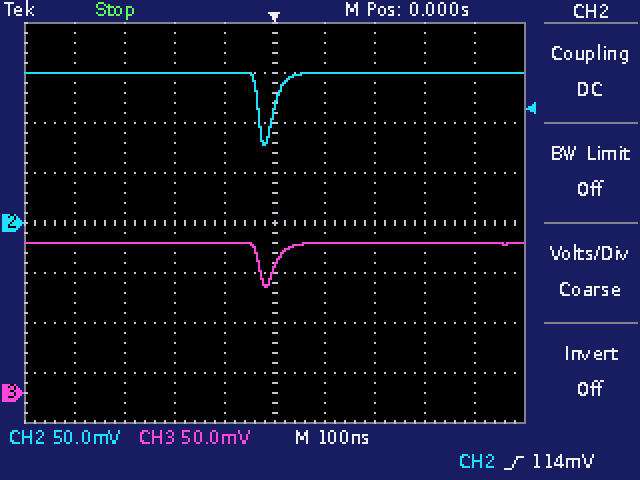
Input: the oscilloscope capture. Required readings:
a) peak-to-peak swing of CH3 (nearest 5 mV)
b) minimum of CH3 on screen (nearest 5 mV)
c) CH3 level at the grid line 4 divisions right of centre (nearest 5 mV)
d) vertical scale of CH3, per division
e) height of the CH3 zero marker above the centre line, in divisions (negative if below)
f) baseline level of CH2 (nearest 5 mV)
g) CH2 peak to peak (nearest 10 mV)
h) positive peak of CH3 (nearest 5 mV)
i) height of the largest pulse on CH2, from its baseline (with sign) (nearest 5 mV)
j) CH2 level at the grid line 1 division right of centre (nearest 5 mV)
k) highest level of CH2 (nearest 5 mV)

45 mV
105 mV
150 mV
50 mV
-3.4 div
150 mV
70 mV
150 mV
-70 mV
150 mV
150 mV
